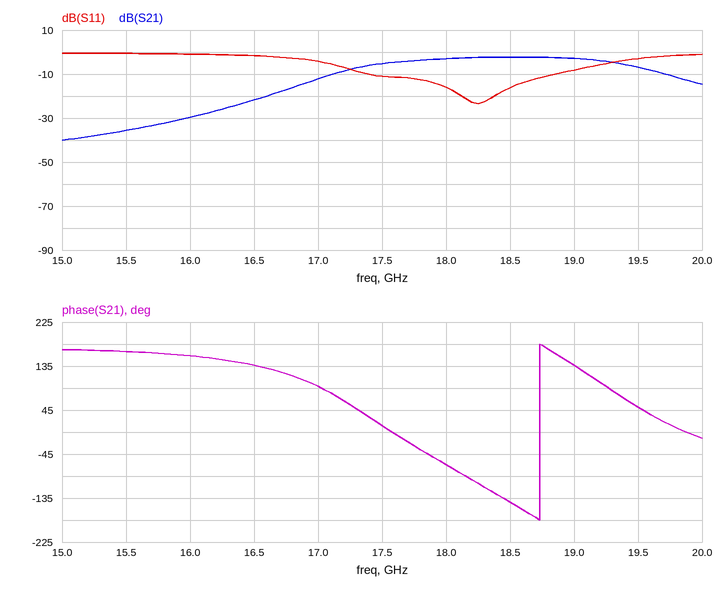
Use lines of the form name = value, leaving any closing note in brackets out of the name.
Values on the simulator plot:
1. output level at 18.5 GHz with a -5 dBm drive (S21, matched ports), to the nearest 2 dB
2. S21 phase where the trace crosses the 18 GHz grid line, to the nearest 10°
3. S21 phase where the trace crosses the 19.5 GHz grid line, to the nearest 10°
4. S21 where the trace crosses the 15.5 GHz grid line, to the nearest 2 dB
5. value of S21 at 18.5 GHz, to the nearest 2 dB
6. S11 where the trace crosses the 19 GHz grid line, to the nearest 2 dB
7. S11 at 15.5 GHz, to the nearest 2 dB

output level at 18.5 GHz with a -5 dBm drive (S21, matched ports), to the nearest 2 dB = -8 dBm
S21 phase where the trace crosses the 18 GHz grid line, to the nearest 10° = -70°
S21 phase where the trace crosses the 19.5 GHz grid line, to the nearest 10° = 50°
S21 where the trace crosses the 15.5 GHz grid line, to the nearest 2 dB = -36 dB
value of S21 at 18.5 GHz, to the nearest 2 dB = -2 dB
S11 where the trace crosses the 19 GHz grid line, to the nearest 2 dB = -8 dB
S11 at 15.5 GHz, to the nearest 2 dB = 0 dB
